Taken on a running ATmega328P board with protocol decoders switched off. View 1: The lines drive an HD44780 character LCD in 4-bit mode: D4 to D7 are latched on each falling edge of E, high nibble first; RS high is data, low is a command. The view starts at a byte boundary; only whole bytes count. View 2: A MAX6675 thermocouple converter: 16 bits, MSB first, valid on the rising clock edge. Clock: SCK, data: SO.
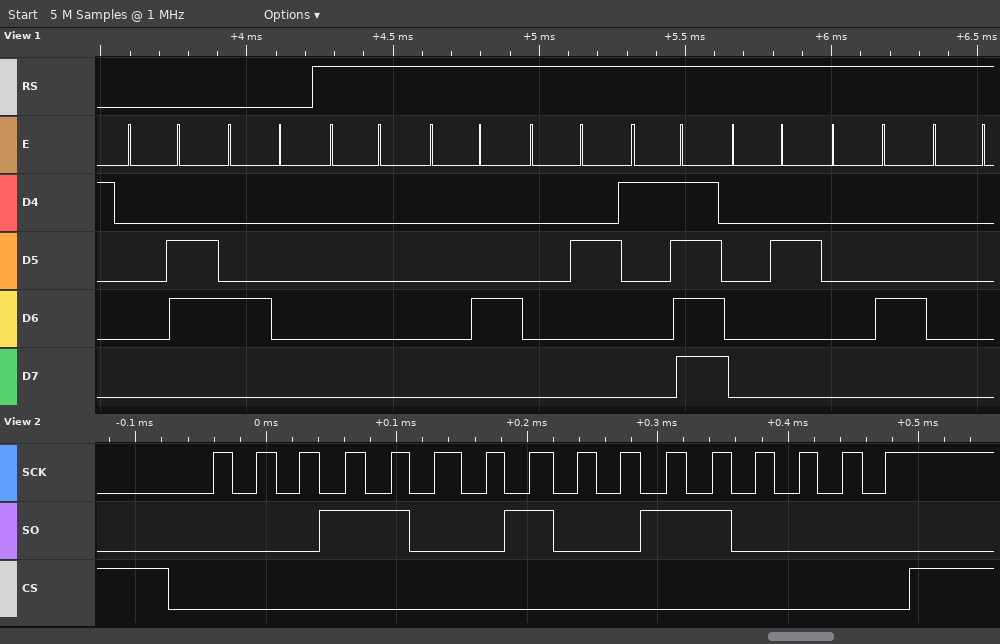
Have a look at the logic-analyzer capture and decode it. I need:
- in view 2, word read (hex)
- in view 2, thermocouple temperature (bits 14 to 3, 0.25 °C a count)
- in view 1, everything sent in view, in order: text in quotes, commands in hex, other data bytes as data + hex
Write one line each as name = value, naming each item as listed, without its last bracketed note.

in view 2, word read = 0x1930
in view 2, thermocouple temperature = 201.50 °C
in view 1, everything sent in view, in order: text in quotes, commands in hex, other data bytes as data + hex = 0x06 0x40 data 00 04 02 1F 02 04 00
